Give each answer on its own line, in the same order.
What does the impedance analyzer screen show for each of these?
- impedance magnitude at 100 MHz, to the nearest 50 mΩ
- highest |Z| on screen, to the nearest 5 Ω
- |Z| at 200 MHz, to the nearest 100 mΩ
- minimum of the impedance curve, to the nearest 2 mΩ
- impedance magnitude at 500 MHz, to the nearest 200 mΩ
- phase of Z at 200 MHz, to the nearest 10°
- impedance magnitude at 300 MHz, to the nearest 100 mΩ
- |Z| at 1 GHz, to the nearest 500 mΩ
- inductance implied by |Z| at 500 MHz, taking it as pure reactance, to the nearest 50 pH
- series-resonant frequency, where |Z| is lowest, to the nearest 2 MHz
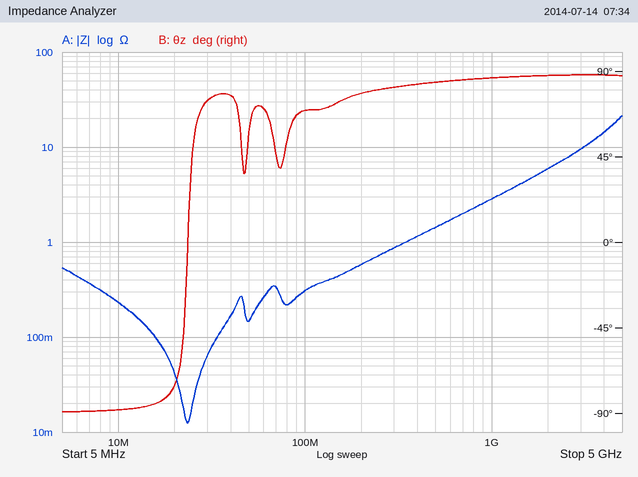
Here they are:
300 mΩ
20 Ω
600 mΩ
12 mΩ
1.4 Ω
80°
900 mΩ
3.0 Ω
450 pH
24 MHz
